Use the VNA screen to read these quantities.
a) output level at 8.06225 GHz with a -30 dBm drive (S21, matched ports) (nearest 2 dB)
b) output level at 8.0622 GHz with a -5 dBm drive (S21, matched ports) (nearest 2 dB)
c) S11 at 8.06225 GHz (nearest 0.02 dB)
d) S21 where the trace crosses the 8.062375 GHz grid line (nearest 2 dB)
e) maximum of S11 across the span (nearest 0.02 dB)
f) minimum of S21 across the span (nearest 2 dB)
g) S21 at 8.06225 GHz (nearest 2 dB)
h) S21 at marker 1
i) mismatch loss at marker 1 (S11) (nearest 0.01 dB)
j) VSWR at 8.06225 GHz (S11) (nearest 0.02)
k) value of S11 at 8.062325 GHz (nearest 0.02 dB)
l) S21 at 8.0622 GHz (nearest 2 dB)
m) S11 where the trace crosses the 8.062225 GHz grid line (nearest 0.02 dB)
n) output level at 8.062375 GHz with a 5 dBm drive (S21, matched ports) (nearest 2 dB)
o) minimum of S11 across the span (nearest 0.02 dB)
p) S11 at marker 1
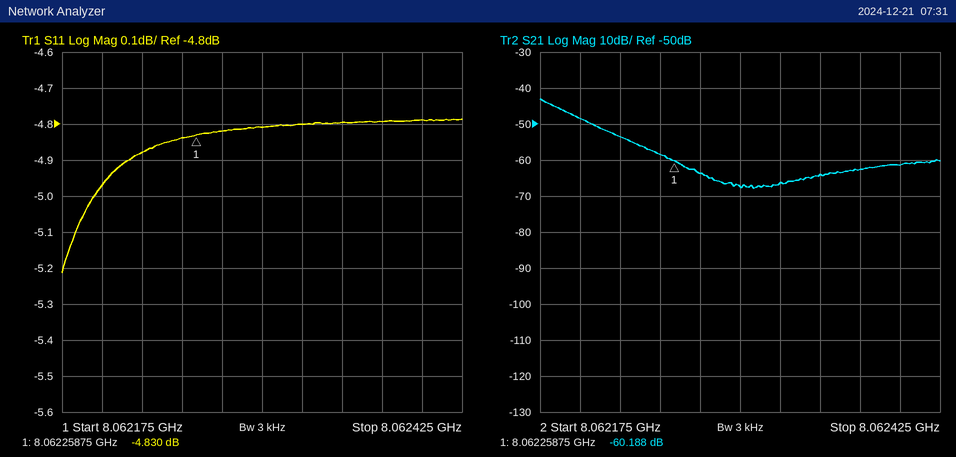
-88 dBm
-54 dBm
-4.84 dB
-62 dB
-4.78 dB
-68 dB
-58 dB
-60.188 dB
1.73 dB
3.68
-4.80 dB
-48 dB
-4.88 dB
-58 dBm
-5.22 dB
-4.830 dB
